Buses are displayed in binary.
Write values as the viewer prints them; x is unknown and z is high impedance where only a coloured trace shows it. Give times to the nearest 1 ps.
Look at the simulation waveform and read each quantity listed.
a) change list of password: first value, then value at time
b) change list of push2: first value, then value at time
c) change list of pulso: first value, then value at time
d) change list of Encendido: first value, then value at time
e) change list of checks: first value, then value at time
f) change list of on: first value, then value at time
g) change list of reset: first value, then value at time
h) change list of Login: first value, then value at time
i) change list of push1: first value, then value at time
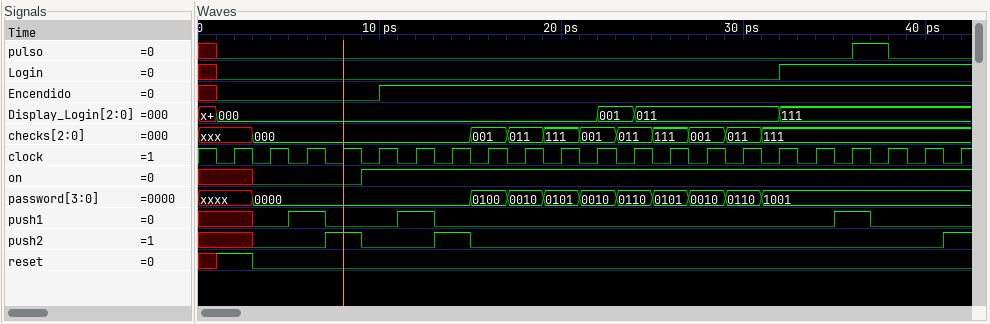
xxxx, 0000 at 3 ps, 0100 at 15 ps, 0010 at 17 ps, 0101 at 19 ps, 0010 at 21 ps, 0110 at 23 ps, 0101 at 25 ps, 0010 at 27 ps, 0110 at 29 ps, 1001 at 31 ps
x, 0 at 3 ps, 1 at 7 ps, 0 at 9 ps, 1 at 13 ps, 0 at 15 ps, 1 at 41 ps
x, 0 at 1 ps, 1 at 36 ps, 0 at 38 ps
x, 0 at 1 ps, 1 at 10 ps
xxx, 000 at 3 ps, 001 at 15 ps, 011 at 17 ps, 111 at 19 ps, 001 at 21 ps, 011 at 23 ps, 111 at 25 ps, 001 at 27 ps, 011 at 29 ps, 111 at 31 ps
x, 0 at 3 ps, 1 at 9 ps
x, 1 at 1 ps, 0 at 3 ps
x, 0 at 1 ps, 1 at 32 ps
x, 0 at 3 ps, 1 at 5 ps, 0 at 7 ps, 1 at 11 ps, 0 at 13 ps, 1 at 35 ps, 0 at 37 ps
